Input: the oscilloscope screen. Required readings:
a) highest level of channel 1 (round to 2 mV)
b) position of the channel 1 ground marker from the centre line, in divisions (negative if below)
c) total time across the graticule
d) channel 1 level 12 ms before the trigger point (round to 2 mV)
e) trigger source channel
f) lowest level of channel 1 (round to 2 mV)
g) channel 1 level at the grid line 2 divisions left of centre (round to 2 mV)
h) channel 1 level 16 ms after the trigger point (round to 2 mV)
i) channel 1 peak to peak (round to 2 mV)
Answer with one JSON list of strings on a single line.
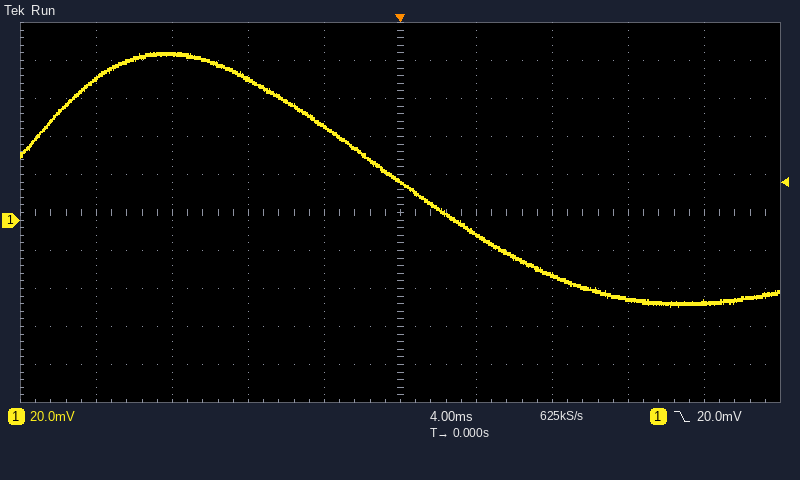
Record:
["88 mV", "-0.2 div", "40 ms", "88 mV", "channel 1", "-46 mV", "74 mV", "-44 mV", "134 mV"]
